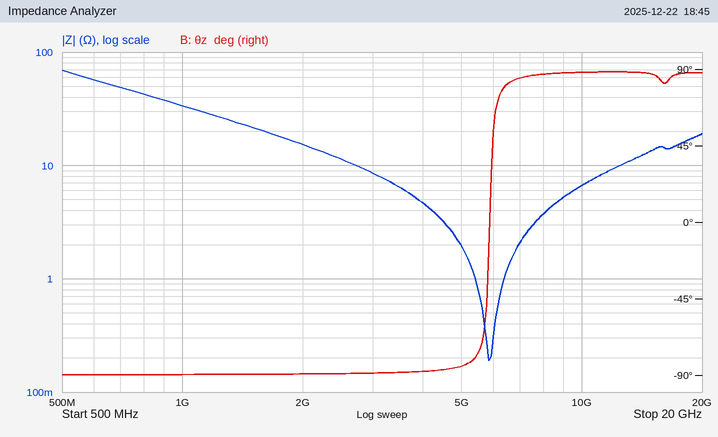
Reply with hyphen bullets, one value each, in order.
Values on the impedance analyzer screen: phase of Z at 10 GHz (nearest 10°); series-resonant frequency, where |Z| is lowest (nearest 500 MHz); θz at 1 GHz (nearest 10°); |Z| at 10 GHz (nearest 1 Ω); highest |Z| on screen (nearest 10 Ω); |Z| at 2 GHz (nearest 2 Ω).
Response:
- 90°
- 6.0 GHz
- -90°
- 7 Ω
- 70 Ω
- 16 Ω
